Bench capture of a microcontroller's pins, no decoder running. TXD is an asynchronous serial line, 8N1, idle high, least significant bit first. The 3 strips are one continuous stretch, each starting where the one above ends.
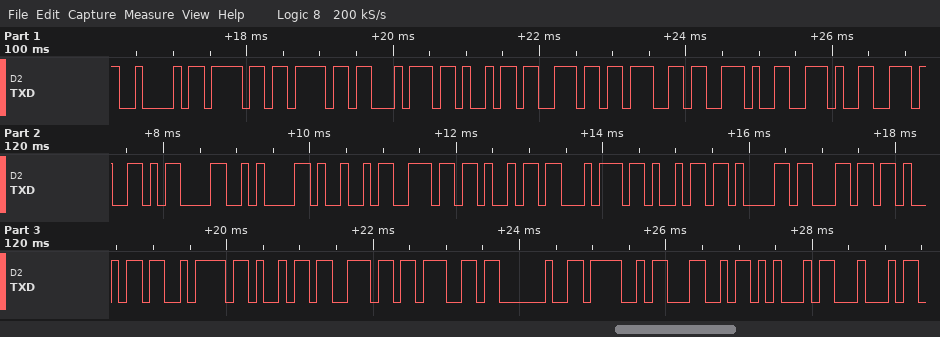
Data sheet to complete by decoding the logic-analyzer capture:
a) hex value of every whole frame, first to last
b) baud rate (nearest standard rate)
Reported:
42 6F 6F 74 69 6E 67 2E 2E 2E 0D 0A 49 6E 69 74 69 61 6C 69 7A 69 6E 67 20 4F 4C 45 44
9600 baud
